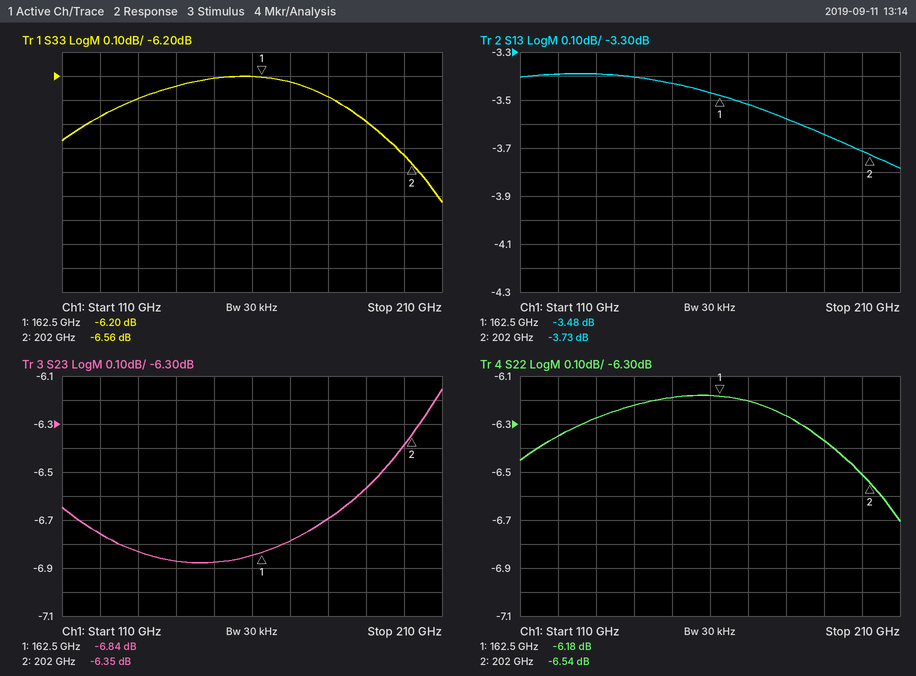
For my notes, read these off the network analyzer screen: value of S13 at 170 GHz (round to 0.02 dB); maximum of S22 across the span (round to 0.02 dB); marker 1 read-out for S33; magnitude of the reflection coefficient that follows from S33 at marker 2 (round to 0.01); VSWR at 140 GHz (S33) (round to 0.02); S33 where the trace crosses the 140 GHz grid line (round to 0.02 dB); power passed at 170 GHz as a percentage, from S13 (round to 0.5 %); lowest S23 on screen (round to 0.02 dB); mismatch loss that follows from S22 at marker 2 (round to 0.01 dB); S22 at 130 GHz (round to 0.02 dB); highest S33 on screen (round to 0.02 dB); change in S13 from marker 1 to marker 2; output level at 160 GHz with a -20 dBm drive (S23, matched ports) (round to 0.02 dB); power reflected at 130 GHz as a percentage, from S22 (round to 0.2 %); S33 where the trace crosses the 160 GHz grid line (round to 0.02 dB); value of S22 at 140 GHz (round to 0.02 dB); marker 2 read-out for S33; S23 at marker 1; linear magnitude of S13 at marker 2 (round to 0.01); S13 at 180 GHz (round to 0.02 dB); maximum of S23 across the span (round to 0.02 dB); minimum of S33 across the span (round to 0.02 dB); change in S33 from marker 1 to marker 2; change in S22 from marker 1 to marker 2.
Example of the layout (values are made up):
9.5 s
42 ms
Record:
-3.52 dB
-6.18 dB
-6.20 dB
0.47
2.90
-6.24 dB
44.5 %
-6.88 dB
1.09 dB
-6.28 dB
-6.20 dB
-0.25 dB
-26.84 dBm
23.6 %
-6.20 dB
-6.22 dB
-6.56 dB
-6.84 dB
0.65
-3.58 dB
-6.16 dB
-6.72 dB
-0.36 dB
-0.36 dB
